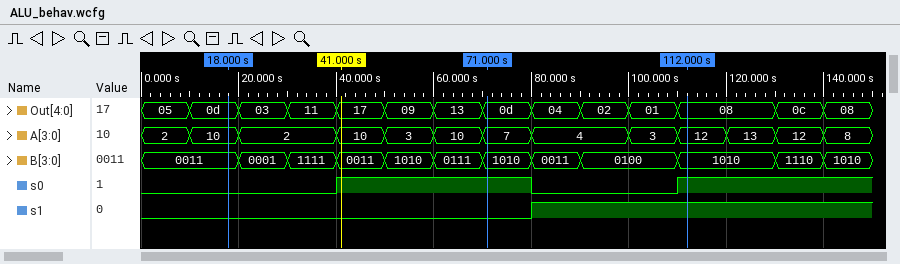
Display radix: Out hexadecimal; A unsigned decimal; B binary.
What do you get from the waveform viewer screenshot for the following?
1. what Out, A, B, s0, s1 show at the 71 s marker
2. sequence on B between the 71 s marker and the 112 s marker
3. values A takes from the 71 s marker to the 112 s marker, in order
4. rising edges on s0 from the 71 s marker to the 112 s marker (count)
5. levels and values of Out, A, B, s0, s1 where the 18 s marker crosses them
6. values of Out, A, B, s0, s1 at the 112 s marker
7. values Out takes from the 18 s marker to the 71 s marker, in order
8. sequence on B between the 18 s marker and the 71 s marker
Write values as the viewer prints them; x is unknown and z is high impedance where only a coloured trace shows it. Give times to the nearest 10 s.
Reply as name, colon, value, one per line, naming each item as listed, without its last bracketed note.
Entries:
what Out, A, B, s0, s1 show at the 71 s marker: Out=0d, A=7, B=1010, s0=1, s1=0
sequence on B between the 71 s marker and the 112 s marker: 1010, 0011, 0100, 1010
values A takes from the 71 s marker to the 112 s marker, in order: 7, 4, 3, 12
rising edges on s0 from the 71 s marker to the 112 s marker: 1
levels and values of Out, A, B, s0, s1 where the 18 s marker crosses them: Out=0d, A=10, B=0011, s0=0, s1=0
values of Out, A, B, s0, s1 at the 112 s marker: Out=08, A=12, B=1010, s0=1, s1=1
values Out takes from the 18 s marker to the 71 s marker, in order: 0d, 03, 11, 17, 09, 13, 0d
sequence on B between the 18 s marker and the 71 s marker: 0011, 0001, 1111, 0011, 1010, 0111, 1010
